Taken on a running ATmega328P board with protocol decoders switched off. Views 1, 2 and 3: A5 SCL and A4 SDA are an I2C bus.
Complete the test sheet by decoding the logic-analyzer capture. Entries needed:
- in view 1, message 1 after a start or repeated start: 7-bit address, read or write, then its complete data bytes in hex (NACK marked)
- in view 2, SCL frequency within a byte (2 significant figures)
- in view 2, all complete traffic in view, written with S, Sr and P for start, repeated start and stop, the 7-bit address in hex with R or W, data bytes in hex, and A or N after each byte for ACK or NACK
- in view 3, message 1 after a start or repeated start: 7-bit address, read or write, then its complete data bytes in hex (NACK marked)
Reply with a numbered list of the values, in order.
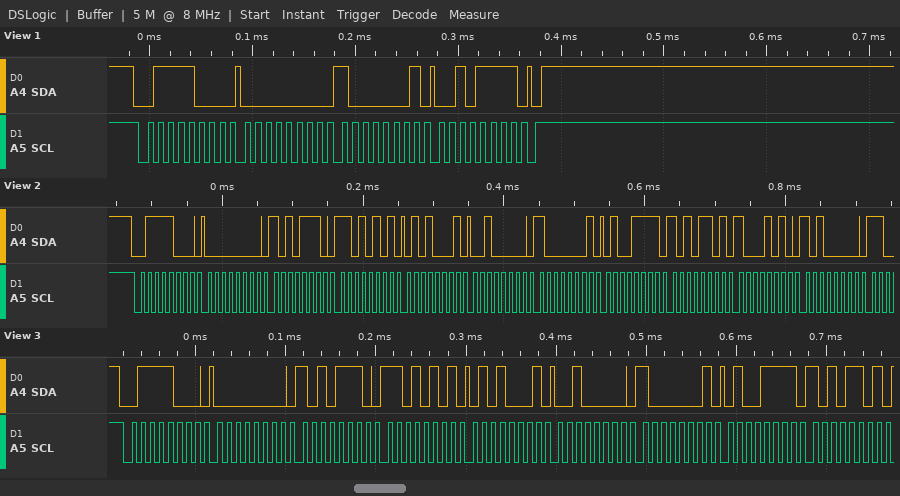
1. 0x3C write: 00 81 2F
2. 100 kHz
3. S 3CW A 00 A AE A D5 A 51 A 20 A 81 A 4F A AD A 8A A A0 A
4. 0x3C write: 00 AE D5 51 20 81 4F AD
